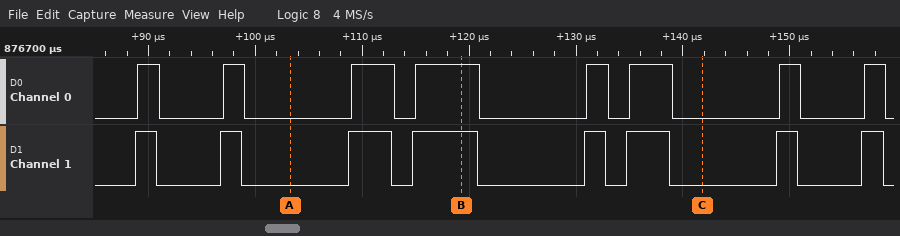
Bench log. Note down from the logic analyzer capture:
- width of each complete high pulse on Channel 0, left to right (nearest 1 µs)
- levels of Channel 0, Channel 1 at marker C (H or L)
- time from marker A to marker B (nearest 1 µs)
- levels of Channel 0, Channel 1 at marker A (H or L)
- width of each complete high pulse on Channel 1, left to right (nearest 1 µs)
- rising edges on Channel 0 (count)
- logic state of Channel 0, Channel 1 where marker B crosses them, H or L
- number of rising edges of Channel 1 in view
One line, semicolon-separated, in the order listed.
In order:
2 µs, 2 µs, 4 µs, 6 µs, 2 µs, 4 µs, 2 µs, 2 µs; Channel 0=L, Channel 1=L; 16 µs; Channel 0=L, Channel 1=L; 2 µs, 2 µs, 4 µs, 6 µs, 2 µs, 4 µs, 2 µs, 2 µs; 8; Channel 0=H, Channel 1=H; 8
